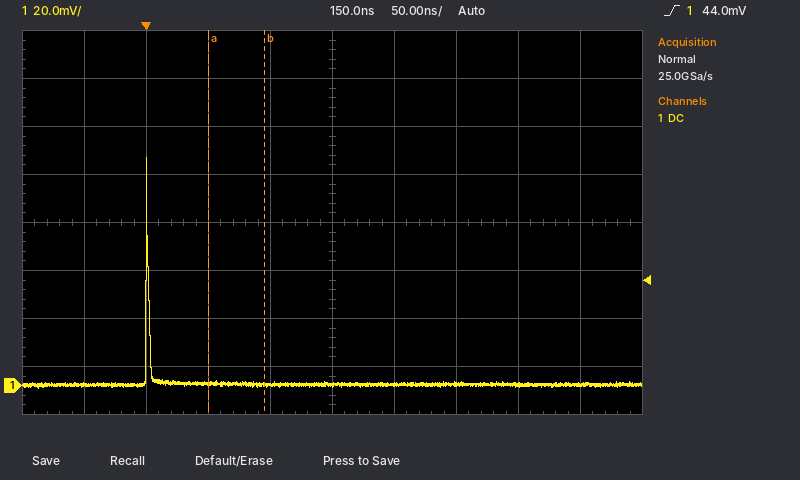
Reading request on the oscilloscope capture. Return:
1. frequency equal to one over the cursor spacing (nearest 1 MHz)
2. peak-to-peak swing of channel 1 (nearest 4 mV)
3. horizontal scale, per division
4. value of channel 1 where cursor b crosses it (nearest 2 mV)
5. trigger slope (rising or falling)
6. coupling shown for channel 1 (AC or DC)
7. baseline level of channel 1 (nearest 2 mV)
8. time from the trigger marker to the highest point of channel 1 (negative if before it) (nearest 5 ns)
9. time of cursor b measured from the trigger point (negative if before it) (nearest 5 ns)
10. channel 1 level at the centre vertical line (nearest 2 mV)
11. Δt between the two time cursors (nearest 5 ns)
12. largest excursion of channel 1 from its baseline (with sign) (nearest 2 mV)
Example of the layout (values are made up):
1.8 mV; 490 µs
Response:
22 MHz; 96 mV; 50 ns; 0 mV; rising; DC; 0 mV; 0 ns; +95 ns; 0 mV; 45 ns; +94 mV
